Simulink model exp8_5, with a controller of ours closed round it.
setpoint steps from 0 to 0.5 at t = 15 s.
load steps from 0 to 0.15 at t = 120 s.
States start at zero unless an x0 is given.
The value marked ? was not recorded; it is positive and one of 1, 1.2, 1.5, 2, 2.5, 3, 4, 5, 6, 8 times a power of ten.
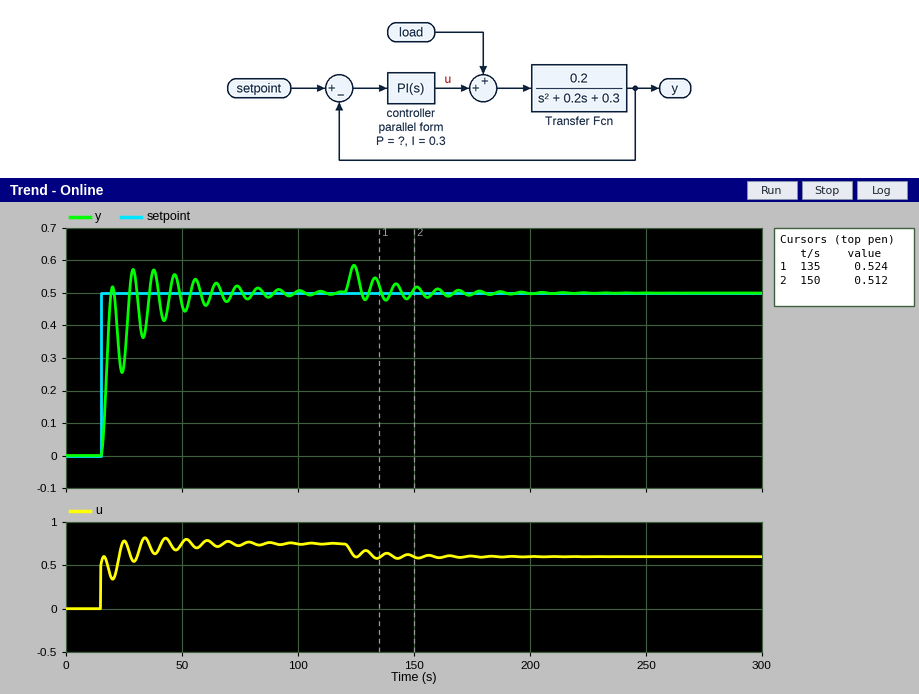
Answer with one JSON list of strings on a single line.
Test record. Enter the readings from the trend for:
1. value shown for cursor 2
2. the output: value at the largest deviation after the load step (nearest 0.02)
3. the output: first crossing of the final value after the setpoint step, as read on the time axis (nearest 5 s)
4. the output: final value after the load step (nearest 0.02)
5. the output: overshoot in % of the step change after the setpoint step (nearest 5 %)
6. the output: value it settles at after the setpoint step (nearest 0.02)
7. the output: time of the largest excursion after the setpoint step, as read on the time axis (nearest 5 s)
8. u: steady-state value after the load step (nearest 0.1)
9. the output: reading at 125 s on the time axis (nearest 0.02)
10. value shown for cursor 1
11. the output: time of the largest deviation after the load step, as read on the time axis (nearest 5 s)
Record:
["0.512", "0.58", "20 s", "0.50", "15 %", "0.50", "30 s", "0.6", "0.58", "0.524", "125 s"]
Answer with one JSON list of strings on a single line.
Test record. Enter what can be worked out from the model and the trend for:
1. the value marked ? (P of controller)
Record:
["1"]
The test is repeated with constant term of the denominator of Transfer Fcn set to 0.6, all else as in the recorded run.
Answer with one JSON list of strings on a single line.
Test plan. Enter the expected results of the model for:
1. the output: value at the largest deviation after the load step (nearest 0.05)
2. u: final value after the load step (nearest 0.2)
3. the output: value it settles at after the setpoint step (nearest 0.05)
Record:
["0.55", "1.4", "0.50"]
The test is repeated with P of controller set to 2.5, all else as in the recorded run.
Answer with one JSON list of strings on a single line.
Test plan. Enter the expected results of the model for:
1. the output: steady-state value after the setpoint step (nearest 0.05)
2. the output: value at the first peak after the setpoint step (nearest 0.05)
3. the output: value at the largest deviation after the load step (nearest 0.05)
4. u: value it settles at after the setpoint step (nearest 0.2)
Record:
["0.50", "0.60", "0.55", "0.8"]
